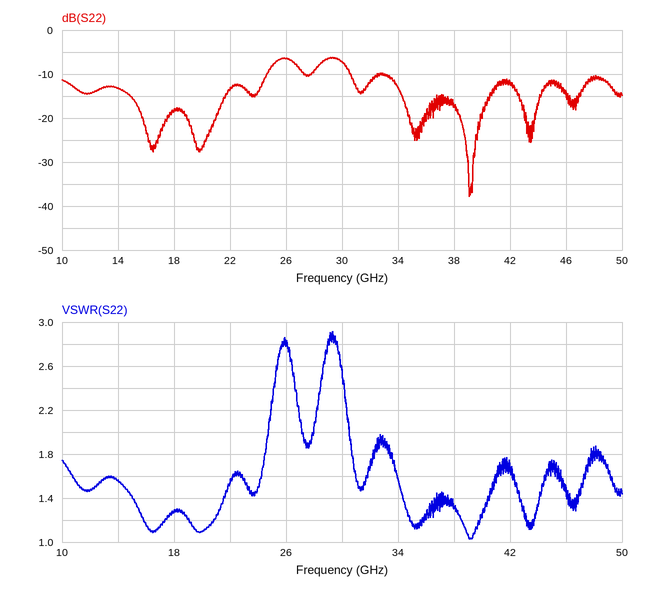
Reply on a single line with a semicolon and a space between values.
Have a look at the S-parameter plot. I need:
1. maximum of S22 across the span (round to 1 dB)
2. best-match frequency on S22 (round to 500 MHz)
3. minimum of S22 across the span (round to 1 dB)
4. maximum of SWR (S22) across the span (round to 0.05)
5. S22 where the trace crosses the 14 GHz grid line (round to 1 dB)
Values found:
-6 dB; 39.0 GHz; -38 dB; 2.90; -13 dB
